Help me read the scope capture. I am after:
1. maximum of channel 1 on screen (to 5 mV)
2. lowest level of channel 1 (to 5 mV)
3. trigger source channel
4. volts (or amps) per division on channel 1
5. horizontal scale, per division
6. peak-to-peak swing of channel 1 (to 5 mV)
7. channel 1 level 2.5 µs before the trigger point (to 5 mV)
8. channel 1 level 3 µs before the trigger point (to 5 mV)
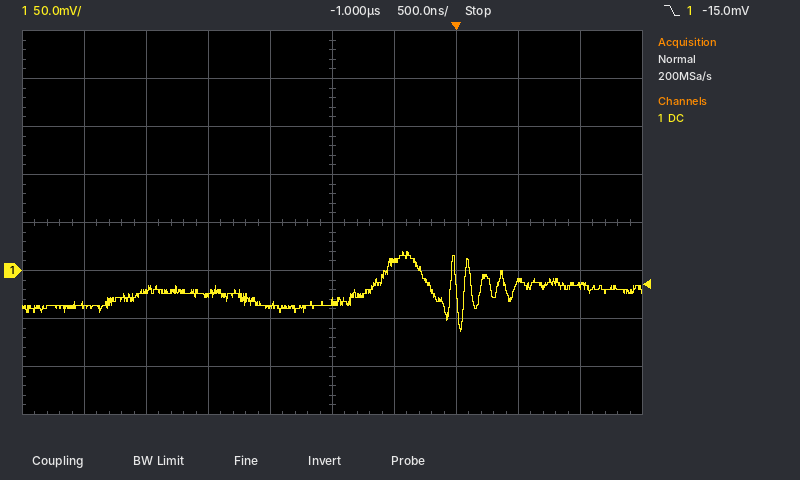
20 mV
-65 mV
channel 1
50 mV
500 ns
85 mV
-20 mV
-35 mV
